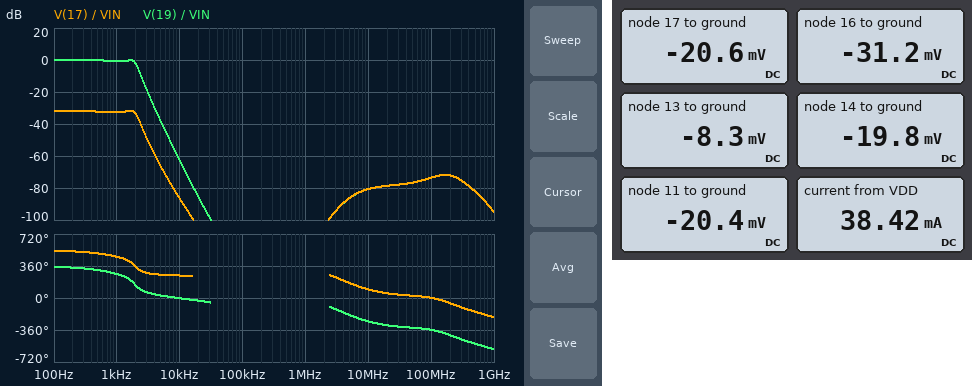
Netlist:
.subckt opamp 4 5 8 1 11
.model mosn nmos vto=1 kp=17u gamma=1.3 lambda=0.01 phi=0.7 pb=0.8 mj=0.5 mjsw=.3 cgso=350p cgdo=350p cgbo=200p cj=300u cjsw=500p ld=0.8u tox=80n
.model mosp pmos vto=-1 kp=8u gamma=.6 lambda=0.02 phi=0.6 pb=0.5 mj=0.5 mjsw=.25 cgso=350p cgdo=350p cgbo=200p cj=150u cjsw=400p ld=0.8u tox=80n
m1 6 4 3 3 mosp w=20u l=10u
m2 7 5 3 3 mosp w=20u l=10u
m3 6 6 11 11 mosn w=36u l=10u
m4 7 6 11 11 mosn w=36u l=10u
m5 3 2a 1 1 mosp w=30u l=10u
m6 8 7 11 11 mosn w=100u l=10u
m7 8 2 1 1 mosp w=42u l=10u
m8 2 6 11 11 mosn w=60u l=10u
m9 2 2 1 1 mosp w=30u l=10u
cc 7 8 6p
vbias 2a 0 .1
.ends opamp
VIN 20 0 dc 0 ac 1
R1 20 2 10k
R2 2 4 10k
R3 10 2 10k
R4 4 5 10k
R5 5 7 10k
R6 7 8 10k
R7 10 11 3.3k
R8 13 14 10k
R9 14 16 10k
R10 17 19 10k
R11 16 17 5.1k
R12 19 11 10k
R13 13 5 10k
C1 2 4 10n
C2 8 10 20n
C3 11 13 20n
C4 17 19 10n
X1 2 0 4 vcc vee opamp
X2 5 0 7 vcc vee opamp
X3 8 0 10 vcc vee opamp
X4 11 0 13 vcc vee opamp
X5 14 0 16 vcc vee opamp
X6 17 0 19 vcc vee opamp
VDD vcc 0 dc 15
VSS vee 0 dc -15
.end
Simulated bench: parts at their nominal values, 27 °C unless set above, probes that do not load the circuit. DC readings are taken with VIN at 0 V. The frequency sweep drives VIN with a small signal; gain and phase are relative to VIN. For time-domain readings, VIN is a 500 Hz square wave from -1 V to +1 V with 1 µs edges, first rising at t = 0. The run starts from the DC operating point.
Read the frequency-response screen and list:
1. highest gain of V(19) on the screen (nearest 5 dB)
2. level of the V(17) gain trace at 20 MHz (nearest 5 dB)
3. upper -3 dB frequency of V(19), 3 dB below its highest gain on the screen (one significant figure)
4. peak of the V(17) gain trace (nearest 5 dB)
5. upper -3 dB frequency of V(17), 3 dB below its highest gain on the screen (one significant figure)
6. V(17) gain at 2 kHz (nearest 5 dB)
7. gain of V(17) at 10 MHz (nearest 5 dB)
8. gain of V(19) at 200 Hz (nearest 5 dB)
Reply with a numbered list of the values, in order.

1. 0 dB
2. -80 dB
3. 2 kHz
4. -30 dB
5. 2 kHz
6. -35 dB
7. -80 dB
8. 0 dB
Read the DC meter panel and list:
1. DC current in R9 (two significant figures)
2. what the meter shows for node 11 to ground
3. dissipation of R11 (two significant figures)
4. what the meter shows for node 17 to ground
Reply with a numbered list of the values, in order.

1. 1.1 µA
2. -20.4 mV
3. 22 nW
4. -20.6 mV
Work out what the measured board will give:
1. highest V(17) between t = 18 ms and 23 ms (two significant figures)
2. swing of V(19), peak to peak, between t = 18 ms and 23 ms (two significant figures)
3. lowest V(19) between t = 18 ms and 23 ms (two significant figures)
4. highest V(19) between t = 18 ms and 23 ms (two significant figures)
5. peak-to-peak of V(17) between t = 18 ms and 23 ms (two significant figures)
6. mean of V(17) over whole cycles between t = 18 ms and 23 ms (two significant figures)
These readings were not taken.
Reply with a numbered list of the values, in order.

1. 9.1 mV
2. 2.4 V
3. -1.2 V
4. 1.2 V
5. 61 mV
6. -21 mV
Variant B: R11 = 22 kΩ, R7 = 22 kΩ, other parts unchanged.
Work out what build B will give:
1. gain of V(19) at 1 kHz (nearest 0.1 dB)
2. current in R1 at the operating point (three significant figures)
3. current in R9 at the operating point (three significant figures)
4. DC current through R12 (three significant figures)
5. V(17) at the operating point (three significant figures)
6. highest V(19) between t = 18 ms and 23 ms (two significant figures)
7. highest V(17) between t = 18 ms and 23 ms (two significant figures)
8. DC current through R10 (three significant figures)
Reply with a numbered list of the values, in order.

1. -18.9 dB
2. 1.99 µA
3. 940 nA
4. 427 nA
5. -20.2 mV
6. 210 mV
7. -15 mV
8. 414 nA
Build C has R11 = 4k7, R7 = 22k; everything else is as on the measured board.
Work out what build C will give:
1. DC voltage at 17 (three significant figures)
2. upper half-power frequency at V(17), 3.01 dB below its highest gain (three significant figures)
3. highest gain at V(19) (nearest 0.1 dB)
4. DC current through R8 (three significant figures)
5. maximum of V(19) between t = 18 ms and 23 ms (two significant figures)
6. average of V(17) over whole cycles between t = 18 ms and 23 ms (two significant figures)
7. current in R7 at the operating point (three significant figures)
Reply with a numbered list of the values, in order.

1. -20.3 mV
2. 1.34 kHz
3. -9.2 dB
4. 367 nA
5. 390 mV
6. -20 mV
7. 710 nA
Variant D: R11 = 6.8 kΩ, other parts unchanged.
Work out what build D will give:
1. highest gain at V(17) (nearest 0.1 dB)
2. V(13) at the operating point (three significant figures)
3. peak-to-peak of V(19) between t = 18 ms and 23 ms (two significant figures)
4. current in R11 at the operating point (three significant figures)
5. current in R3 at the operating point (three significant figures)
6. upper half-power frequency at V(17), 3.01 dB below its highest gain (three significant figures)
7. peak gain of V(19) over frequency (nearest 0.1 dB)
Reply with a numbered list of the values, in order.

1. -32.4 dB
2. -7.23 mV
3. 2.1 V
4. 1.73 µA
5. 632 nA
6. 1.97 kHz
7. -0.9 dB
